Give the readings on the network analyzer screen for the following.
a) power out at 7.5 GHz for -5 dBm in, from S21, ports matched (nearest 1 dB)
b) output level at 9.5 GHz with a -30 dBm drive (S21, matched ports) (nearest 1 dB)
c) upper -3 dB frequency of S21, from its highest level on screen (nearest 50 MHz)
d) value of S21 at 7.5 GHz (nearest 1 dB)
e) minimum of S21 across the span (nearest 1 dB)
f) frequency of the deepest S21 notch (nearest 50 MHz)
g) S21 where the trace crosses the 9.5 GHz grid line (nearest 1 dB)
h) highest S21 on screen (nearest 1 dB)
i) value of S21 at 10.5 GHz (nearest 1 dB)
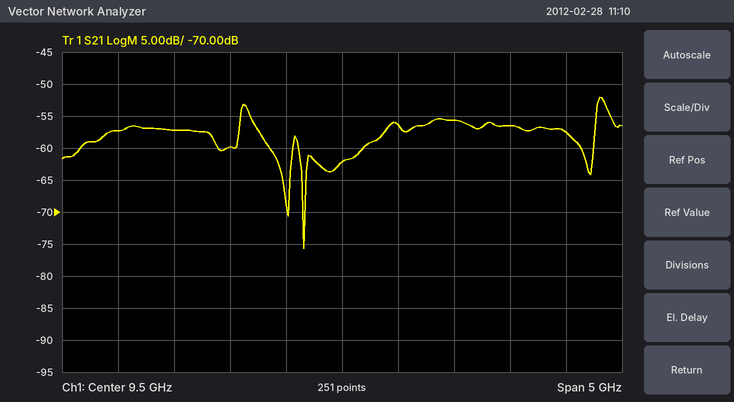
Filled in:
-62 dBm
-92 dBm
11.90 GHz
-57 dB
-76 dB
9.15 GHz
-62 dB
-52 dB
-56 dB
